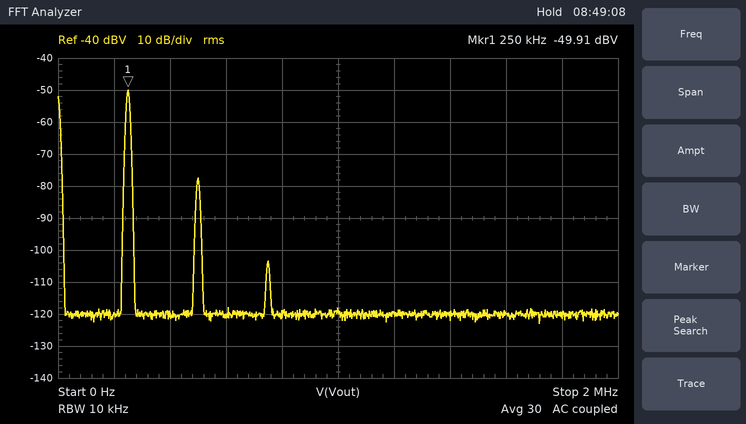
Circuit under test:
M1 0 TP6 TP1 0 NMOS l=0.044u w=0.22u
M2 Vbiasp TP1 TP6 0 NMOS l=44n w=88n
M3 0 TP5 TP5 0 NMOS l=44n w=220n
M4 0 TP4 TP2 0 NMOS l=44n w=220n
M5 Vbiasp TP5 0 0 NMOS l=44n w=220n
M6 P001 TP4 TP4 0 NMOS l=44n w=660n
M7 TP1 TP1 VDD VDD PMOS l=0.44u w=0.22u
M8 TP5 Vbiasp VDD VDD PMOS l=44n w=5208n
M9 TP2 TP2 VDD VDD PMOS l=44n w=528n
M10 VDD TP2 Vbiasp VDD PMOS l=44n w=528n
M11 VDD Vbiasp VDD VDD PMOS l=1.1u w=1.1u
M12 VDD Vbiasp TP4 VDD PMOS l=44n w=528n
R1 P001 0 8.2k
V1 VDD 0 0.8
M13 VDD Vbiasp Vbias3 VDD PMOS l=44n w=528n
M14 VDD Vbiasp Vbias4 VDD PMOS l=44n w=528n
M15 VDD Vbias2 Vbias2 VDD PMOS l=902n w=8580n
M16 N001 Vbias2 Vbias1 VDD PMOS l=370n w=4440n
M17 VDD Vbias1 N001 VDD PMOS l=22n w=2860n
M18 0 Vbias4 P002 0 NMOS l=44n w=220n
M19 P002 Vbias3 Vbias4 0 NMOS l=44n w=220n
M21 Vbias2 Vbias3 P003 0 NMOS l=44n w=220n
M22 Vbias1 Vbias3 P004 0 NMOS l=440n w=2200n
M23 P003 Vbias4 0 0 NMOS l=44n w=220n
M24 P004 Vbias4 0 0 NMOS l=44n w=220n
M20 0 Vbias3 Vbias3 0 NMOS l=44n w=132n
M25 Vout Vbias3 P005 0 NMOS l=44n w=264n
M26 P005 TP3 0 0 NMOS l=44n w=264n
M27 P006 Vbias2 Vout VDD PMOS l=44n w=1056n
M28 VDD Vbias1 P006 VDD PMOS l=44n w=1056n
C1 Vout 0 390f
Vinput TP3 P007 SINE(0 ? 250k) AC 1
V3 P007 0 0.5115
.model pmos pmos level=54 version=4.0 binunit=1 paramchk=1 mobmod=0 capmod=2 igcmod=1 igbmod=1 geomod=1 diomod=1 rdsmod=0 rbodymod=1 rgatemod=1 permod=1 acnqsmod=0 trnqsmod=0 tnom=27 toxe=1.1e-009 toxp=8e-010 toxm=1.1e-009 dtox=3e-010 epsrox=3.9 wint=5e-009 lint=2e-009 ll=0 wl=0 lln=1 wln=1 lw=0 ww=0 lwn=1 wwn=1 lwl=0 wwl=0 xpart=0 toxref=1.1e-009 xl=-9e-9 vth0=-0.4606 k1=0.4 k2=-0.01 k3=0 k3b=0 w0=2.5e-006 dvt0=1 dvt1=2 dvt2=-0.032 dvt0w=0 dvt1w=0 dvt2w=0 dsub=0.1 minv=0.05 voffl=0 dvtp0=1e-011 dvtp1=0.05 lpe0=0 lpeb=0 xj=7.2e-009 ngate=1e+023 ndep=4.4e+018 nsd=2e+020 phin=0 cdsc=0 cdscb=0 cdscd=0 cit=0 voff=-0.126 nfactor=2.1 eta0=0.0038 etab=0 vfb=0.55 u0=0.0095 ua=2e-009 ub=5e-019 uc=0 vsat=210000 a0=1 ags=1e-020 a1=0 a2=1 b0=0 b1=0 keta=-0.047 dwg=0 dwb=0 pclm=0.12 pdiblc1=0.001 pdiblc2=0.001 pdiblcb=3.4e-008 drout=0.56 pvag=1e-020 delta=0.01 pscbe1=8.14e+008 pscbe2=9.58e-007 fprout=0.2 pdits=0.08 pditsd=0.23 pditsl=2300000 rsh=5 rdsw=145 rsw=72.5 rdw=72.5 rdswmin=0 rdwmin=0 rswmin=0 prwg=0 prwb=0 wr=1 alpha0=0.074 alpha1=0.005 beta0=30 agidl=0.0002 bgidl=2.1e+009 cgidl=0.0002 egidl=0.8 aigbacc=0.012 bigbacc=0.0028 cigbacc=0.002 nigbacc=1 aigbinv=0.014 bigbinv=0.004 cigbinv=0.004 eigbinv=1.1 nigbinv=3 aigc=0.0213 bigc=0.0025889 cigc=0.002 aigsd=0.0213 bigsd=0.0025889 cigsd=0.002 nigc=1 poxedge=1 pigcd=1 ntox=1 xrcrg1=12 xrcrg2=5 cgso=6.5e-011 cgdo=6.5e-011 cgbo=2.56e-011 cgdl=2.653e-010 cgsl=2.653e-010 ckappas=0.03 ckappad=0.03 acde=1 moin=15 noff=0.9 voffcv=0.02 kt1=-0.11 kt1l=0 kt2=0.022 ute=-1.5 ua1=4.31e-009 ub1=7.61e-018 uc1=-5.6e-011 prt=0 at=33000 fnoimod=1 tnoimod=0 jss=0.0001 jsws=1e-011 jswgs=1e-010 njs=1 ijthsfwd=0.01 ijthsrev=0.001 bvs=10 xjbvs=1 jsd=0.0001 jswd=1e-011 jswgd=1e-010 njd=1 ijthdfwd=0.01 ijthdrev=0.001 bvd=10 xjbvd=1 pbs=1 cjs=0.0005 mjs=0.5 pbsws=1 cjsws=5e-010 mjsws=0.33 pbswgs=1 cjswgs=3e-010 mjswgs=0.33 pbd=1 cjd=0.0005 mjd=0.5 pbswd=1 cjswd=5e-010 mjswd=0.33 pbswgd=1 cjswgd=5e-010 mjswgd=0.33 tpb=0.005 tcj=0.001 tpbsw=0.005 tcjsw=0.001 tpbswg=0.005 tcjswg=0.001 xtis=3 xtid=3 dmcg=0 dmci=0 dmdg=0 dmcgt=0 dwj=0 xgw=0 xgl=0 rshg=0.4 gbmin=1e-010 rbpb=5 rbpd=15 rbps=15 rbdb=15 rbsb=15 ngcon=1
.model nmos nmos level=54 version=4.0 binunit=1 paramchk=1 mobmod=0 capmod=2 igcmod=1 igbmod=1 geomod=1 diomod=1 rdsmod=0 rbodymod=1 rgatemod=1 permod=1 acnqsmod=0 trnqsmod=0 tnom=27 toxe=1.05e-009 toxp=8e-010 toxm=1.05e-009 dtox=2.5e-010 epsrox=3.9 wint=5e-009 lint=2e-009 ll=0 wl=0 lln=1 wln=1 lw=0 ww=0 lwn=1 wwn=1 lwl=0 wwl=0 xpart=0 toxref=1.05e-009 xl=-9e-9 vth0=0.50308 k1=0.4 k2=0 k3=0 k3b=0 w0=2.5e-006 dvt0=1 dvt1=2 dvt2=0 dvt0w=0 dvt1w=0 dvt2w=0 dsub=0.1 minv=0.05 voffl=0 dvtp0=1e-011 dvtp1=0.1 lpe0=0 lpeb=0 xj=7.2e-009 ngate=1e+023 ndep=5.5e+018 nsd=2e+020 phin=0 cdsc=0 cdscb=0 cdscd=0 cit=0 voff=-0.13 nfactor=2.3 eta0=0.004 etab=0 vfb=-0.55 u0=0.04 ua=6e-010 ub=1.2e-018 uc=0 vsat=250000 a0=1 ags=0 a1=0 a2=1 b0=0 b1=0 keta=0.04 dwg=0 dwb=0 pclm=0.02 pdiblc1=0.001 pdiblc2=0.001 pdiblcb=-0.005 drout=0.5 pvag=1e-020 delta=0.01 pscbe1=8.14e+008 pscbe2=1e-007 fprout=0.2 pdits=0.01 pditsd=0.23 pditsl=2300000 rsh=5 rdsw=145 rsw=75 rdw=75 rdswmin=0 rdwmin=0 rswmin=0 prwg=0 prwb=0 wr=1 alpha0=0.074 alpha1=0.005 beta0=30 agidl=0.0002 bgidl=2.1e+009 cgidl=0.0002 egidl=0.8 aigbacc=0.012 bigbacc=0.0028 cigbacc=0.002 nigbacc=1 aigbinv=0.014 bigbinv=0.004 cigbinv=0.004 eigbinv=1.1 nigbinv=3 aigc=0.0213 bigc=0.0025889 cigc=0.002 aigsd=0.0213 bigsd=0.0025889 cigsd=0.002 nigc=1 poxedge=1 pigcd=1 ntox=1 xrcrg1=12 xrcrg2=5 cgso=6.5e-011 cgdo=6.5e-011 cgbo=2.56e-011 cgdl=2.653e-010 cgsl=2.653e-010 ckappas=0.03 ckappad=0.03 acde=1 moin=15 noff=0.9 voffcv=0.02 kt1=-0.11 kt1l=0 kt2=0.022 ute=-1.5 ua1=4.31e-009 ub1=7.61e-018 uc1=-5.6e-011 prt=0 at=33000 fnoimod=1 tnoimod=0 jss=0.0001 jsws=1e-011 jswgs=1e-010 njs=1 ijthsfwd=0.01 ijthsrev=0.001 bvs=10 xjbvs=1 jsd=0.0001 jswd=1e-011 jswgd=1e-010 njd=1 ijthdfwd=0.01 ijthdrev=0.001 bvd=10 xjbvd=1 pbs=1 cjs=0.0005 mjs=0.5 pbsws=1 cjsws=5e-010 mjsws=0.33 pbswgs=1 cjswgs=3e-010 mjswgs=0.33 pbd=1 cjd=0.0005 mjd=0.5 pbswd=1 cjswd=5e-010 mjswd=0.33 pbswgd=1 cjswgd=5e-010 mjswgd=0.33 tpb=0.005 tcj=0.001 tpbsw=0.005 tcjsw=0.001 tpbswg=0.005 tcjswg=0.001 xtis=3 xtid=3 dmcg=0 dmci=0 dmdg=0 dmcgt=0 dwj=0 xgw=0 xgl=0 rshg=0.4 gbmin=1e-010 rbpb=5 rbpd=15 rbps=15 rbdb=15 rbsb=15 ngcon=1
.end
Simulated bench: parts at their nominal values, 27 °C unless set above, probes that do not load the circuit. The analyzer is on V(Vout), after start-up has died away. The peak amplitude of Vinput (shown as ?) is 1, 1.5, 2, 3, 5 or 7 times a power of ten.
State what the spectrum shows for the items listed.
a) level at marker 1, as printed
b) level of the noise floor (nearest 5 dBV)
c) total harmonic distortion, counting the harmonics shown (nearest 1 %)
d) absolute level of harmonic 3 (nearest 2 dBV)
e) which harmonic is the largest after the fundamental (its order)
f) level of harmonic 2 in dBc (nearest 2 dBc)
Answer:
-49.91 dBV
-120 dBV
4 %
-104 dBV
2
-28 dBc
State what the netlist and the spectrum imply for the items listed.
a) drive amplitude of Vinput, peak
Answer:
1 mV
